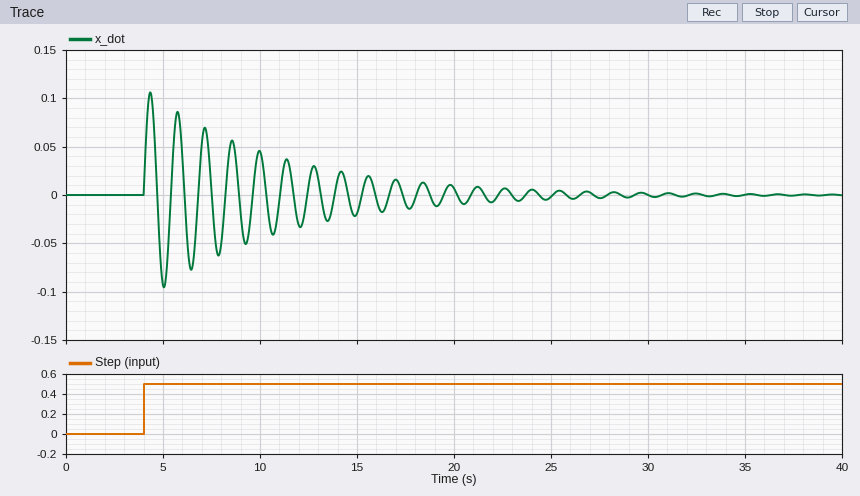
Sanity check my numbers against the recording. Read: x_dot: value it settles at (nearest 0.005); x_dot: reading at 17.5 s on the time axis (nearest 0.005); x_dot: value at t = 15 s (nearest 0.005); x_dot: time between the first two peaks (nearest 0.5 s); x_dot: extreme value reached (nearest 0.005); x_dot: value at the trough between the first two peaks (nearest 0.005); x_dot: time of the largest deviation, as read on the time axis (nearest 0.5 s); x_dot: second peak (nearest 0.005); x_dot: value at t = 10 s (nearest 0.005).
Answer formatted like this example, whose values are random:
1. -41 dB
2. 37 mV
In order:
1. 0.000
2. -0.010
3. -0.020
4. 1.5 s
5. 0.105
6. -0.095
7. 4.5 s
8. 0.085
9. 0.045
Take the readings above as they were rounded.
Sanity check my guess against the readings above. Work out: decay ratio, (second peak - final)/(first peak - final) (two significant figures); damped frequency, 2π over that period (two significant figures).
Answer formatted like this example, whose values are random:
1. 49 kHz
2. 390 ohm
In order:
1. 0.81
2. 4.2 rad/s
